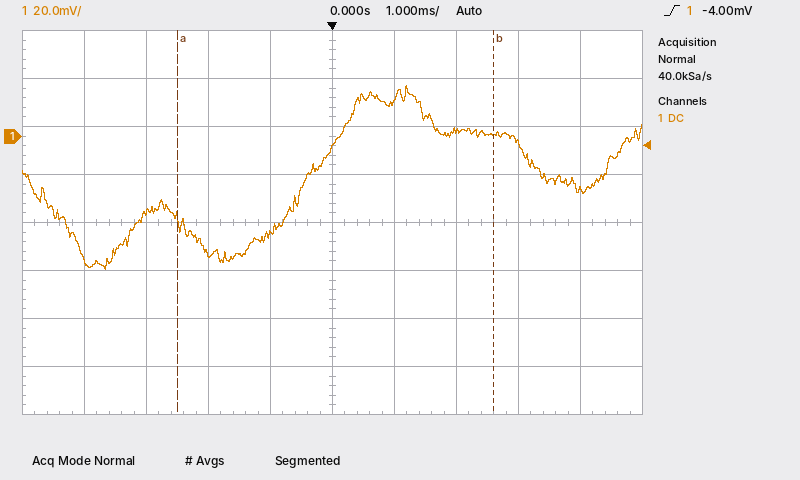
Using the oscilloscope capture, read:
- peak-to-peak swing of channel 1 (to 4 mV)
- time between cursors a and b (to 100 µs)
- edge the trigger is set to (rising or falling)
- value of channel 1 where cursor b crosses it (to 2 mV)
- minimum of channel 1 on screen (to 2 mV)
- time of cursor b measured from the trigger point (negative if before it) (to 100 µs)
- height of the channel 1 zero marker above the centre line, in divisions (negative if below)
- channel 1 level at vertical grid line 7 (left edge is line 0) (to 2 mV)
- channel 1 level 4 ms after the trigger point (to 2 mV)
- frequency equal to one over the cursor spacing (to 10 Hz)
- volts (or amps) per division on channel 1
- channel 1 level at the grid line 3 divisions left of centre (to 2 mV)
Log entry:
76 mV
5.1 ms
rising
0 mV
-56 mV
+2.6 ms
+1.8 div
2 mV
-22 mV
200 Hz
20 mV
-32 mV
